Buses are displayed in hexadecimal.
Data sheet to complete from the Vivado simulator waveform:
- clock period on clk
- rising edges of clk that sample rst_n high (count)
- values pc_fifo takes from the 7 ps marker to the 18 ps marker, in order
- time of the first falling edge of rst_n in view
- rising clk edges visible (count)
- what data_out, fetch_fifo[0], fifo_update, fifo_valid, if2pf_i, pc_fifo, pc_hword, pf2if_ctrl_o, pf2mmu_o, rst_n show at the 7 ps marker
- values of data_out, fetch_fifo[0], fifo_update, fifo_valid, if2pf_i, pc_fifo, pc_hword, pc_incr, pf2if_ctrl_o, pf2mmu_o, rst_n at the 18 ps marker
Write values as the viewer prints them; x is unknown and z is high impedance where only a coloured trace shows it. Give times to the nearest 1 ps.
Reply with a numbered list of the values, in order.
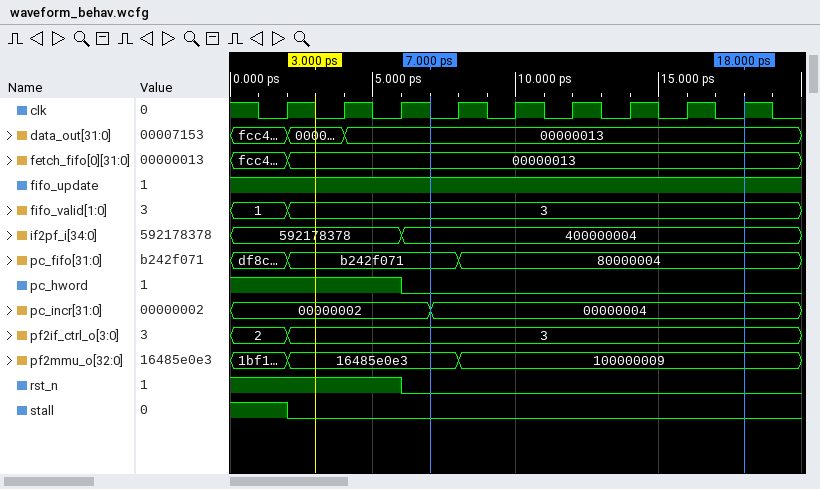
1. 2 ps
2. 3
3. b242f071, 80000004
4. 6 ps
5. 9
6. data_out=00000013, fetch_fifo[0]=00000013, fifo_update=1, fifo_valid=3, if2pf_i=400000004, pc_fifo=b242f071, pc_hword=0, pf2if_ctrl_o=3, pf2mmu_o=16485e0e3, rst_n=0
7. data_out=00000013, fetch_fifo[0]=00000013, fifo_update=1, fifo_valid=3, if2pf_i=400000004, pc_fifo=80000004, pc_hword=0, pc_incr=00000004, pf2if_ctrl_o=3, pf2mmu_o=100000009, rst_n=0
